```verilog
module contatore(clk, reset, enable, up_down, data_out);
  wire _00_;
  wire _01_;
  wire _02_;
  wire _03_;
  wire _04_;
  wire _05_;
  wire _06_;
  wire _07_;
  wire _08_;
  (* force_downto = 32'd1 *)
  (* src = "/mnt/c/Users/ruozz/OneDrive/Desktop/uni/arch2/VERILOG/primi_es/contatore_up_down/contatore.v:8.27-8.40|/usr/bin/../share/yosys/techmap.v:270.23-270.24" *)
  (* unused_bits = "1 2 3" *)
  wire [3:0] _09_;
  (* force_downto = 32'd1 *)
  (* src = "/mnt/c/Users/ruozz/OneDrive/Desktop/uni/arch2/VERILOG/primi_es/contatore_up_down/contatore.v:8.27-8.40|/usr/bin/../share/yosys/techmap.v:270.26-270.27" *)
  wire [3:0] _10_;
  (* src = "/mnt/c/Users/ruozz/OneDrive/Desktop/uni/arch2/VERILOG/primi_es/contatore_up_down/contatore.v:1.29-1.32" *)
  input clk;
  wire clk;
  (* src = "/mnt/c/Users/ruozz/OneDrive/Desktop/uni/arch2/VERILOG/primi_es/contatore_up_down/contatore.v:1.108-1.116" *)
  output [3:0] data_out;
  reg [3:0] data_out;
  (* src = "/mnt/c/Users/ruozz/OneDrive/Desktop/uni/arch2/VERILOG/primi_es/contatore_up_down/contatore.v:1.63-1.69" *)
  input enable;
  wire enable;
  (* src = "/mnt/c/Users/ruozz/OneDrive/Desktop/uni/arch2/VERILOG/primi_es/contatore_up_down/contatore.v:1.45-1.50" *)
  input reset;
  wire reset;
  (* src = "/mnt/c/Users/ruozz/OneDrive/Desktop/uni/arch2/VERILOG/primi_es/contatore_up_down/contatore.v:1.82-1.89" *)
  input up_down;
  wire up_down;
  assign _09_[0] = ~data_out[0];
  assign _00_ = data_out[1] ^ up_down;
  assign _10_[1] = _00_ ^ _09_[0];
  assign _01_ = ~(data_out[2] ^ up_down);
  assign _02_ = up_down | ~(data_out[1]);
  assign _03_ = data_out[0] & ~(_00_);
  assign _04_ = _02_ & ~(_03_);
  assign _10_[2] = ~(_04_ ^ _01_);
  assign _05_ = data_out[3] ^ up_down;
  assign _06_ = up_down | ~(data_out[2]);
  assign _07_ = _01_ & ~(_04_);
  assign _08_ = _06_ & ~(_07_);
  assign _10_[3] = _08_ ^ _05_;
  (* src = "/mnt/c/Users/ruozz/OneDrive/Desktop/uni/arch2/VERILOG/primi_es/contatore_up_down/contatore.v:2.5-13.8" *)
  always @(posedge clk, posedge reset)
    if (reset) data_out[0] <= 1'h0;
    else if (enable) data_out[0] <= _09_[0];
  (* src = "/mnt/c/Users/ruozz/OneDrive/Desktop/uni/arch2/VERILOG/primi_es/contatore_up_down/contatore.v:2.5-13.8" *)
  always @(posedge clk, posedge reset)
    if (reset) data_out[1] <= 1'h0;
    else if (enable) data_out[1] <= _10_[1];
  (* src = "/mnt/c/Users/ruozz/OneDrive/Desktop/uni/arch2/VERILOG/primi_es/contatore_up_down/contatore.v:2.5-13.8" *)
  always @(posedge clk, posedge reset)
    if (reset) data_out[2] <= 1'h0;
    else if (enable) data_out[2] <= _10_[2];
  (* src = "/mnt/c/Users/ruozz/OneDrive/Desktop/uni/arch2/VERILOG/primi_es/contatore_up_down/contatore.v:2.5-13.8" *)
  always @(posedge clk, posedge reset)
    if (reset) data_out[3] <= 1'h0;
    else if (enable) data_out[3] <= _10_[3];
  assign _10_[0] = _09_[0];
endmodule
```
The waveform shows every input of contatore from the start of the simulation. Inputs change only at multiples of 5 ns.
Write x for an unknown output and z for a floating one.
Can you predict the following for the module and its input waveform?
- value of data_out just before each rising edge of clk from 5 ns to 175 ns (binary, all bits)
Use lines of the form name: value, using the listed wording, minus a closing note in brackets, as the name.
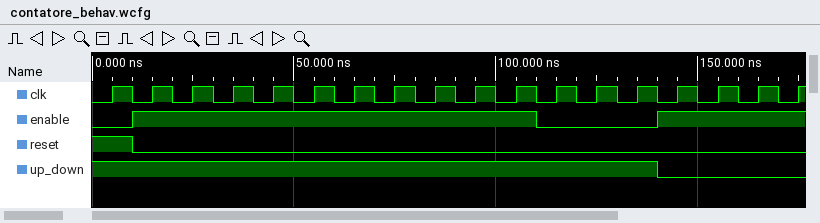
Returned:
value of data_out just before each rising edge of clk from 5 ns to 175 ns: 0000, 0000, 0001, 0010, 0011, 0100, 0101, 0110, 0111, 1000, 1001, 1010, 1010, 1010, 1010, 1001, 1000, 0111
